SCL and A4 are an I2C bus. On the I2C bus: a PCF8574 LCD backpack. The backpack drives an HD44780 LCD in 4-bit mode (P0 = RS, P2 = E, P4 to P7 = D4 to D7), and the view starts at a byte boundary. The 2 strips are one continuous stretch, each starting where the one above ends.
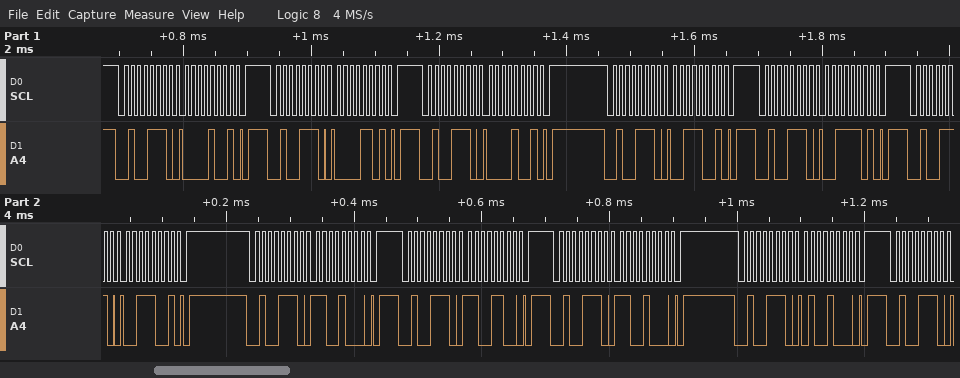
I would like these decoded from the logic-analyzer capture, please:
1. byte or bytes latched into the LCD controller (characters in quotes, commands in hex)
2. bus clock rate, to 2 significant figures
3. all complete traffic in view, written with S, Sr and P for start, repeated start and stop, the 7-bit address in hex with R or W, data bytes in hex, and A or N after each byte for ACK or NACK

data 0x03
100 kHz
S 27W A 09 A P S 27W A 0D A P S 27W A 09 A P S 27W A 39 A P S 27W A 3D A P S 27W A 39 A P S 27W A C8 A P S 27W A CC A P S 27W A C8 A P S 27W A 48 A P S 27W A
